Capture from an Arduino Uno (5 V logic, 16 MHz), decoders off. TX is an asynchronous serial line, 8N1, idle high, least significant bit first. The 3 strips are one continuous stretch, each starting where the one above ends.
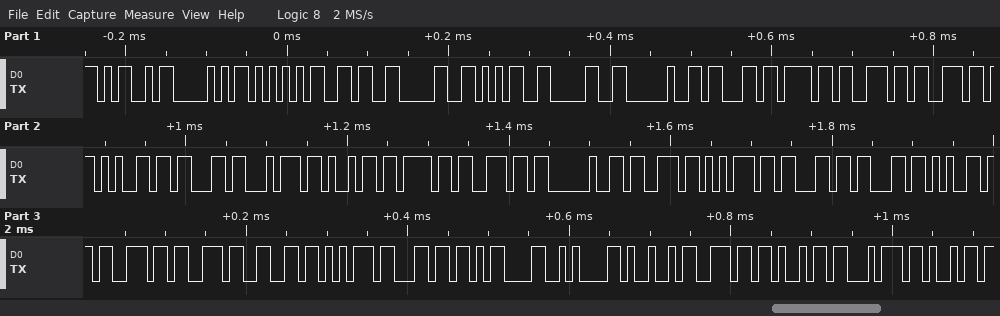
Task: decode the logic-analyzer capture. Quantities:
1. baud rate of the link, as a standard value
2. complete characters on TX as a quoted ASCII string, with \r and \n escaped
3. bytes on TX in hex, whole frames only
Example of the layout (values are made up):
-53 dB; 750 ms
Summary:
115200 baud; "MPU6050 connection successful\r\nIniti"; 0x4D 0x50 0x55 0x36 0x30 0x35 0x30 0x20 0x63 0x6F 0x6E 0x6E 0x65 0x63 0x74 0x69 0x6F 0x6E 0x20 0x73 0x75 0x63 0x63 0x65 0x73 0x73 0x66 0x75 0x6C 0x0D 0x0A 0x49 0x6E 0x69 0x74 0x69
